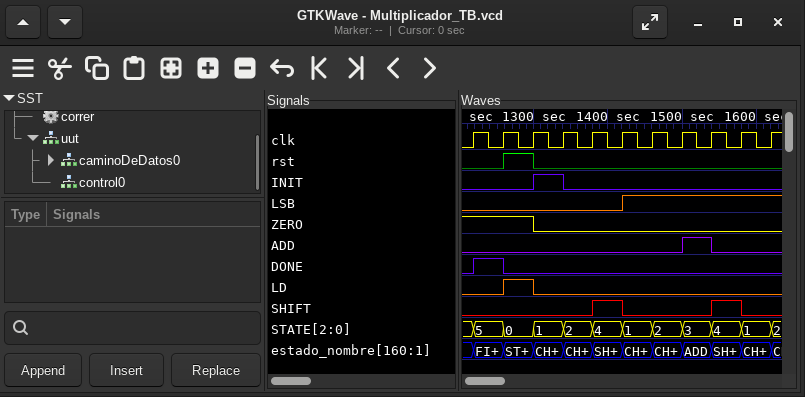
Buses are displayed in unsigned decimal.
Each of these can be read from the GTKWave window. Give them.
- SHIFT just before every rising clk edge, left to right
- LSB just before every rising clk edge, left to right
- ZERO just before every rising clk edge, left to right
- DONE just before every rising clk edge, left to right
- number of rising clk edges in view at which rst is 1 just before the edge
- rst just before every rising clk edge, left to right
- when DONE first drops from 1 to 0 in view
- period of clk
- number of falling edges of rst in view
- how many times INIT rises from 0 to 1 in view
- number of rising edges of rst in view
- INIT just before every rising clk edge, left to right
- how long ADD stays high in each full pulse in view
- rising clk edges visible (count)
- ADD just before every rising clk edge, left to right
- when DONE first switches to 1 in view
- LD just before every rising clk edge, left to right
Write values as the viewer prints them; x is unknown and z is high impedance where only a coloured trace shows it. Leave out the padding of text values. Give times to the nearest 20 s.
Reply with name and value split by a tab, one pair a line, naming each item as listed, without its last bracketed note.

SHIFT just before every rising clk edge, left to right	0 0 0 0 0 1 0 0 0 1 0
LSB just before every rising clk edge, left to right	0 0 0 0 0 0 1 1 1 1 1
ZERO just before every rising clk edge, left to right	1 1 1 0 0 0 0 0 0 0 0
DONE just before every rising clk edge, left to right	0 1 0 0 0 0 0 0 0 0 0
number of rising clk edges in view at which rst is 1 just before the edge	1
rst just before every rising clk edge, left to right	0 0 1 0 0 0 0 0 0 0 0
when DONE first drops from 1 to 0 in view	1260 s
period of clk	40 s
number of falling edges of rst in view	1
how many times INIT rises from 0 to 1 in view	1
number of rising edges of rst in view	1
INIT just before every rising clk edge, left to right	0 0 0 1 0 0 0 0 0 0 0
how long ADD stays high in each full pulse in view	40 s
rising clk edges visible	11
ADD just before every rising clk edge, left to right	0 0 0 0 0 0 0 0 1 0 0
when DONE first switches to 1 in view	1220 s
LD just before every rising clk edge, left to right	0 0 1 0 0 0 0 0 0 0 0
